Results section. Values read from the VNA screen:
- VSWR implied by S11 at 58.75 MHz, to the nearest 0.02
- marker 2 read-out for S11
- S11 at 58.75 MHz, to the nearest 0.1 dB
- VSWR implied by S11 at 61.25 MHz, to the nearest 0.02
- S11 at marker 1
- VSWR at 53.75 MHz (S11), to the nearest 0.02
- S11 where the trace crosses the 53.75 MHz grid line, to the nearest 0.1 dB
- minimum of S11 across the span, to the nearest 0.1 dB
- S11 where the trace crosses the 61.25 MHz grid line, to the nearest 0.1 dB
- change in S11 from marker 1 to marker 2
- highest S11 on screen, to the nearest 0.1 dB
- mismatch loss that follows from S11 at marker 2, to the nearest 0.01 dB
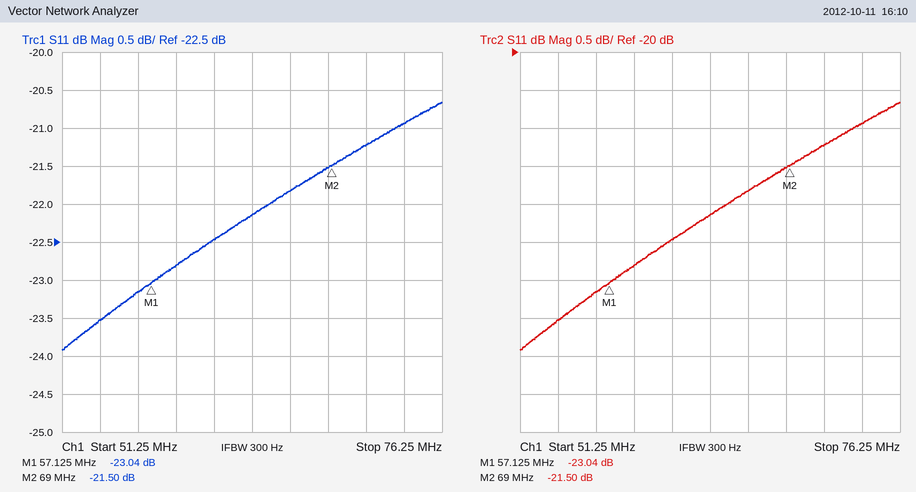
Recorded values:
1.16
-21.50 dB
-22.8 dB
1.16
-23.04 dB
1.14
-23.5 dB
-23.9 dB
-22.5 dB
1.54 dB
-20.7 dB
0.03 dB
